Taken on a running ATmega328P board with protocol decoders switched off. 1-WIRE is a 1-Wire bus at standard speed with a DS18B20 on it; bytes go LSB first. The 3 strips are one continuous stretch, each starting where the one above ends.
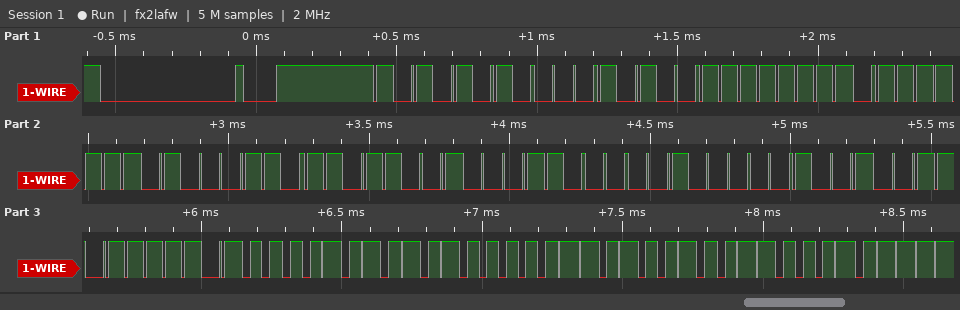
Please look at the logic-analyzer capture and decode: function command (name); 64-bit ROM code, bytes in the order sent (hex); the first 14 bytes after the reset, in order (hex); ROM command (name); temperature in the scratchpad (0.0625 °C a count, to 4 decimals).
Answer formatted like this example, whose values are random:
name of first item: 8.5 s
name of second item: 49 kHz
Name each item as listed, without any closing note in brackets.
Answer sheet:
function command: Read Scratchpad
64-bit ROM code, bytes in the order sent: 28 FF FE 62 9B 18 04 C9
the first 14 bytes after the reset, in order: 55 28 FF FE 62 9B 18 04 C9 BE 50 05 4B 46
ROM command: Match ROM
temperature in the scratchpad: 85.0000 °C
